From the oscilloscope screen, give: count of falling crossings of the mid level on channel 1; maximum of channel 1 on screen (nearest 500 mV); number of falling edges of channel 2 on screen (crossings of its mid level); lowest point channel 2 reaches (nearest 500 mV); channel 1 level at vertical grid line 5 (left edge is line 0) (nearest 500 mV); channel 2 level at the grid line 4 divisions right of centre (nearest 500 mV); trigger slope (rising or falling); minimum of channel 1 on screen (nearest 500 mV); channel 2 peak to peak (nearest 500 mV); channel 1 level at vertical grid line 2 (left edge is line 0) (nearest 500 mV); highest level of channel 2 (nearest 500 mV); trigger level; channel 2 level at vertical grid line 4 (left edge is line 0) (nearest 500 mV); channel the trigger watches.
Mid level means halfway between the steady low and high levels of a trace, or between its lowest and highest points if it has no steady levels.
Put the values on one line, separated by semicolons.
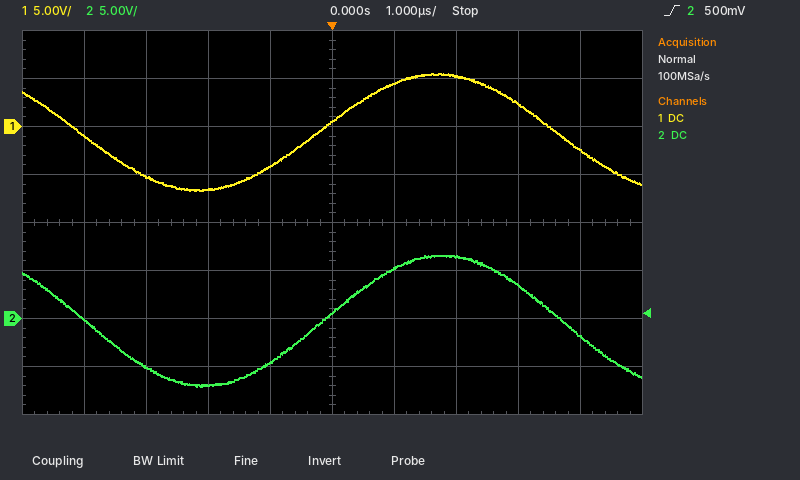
2; 5.5 V; 2; -7.0 V; 500 mV; -2.0 V; rising; -6.5 V; 13.5 V; -5.0 V; 6.5 V; 500 mV; -4.5 V; channel 2
